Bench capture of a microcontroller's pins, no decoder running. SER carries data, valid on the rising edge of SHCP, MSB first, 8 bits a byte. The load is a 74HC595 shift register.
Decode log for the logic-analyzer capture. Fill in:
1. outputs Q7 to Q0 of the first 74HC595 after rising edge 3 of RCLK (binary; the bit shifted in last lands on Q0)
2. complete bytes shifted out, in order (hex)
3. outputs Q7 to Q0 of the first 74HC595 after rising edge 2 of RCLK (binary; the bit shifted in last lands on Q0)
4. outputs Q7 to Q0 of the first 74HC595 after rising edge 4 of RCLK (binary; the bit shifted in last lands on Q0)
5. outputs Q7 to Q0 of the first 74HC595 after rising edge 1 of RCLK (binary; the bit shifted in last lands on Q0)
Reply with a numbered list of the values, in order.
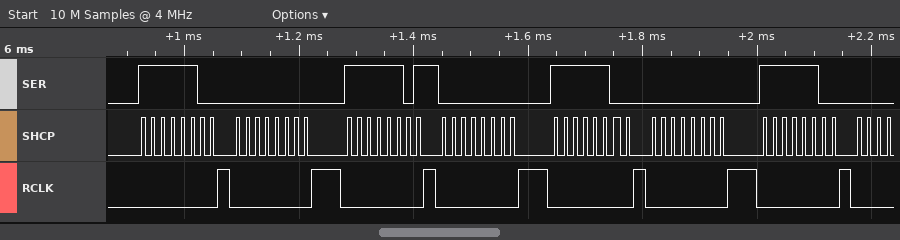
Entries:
1. 11111101
2. FC 00 FD 00 FC 00 FC
3. 00000000
4. 00000000
5. 11111100
